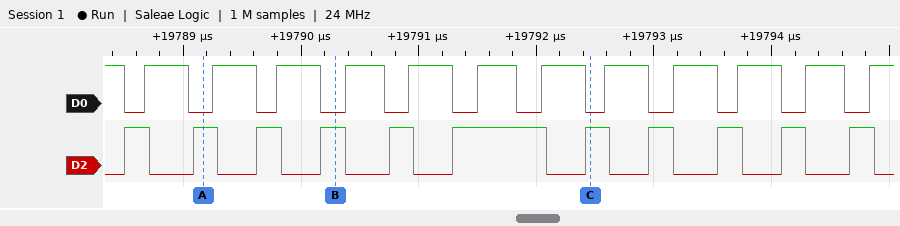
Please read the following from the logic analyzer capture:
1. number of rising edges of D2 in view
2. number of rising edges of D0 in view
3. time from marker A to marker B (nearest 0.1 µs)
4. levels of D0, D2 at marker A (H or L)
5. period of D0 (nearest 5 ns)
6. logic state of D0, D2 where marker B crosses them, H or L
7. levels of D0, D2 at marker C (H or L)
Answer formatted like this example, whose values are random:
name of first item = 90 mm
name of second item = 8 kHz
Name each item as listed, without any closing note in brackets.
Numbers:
number of rising edges of D2 in view = 11
number of rising edges of D0 in view = 12
time from marker A to marker B = 1.1 µs
levels of D0, D2 at marker A = D0=L, D2=H
period of D0 = 560 ns
logic state of D0, D2 where marker B crosses them, H or L = D0=L, D2=H
levels of D0, D2 at marker C = D0=L, D2=H
